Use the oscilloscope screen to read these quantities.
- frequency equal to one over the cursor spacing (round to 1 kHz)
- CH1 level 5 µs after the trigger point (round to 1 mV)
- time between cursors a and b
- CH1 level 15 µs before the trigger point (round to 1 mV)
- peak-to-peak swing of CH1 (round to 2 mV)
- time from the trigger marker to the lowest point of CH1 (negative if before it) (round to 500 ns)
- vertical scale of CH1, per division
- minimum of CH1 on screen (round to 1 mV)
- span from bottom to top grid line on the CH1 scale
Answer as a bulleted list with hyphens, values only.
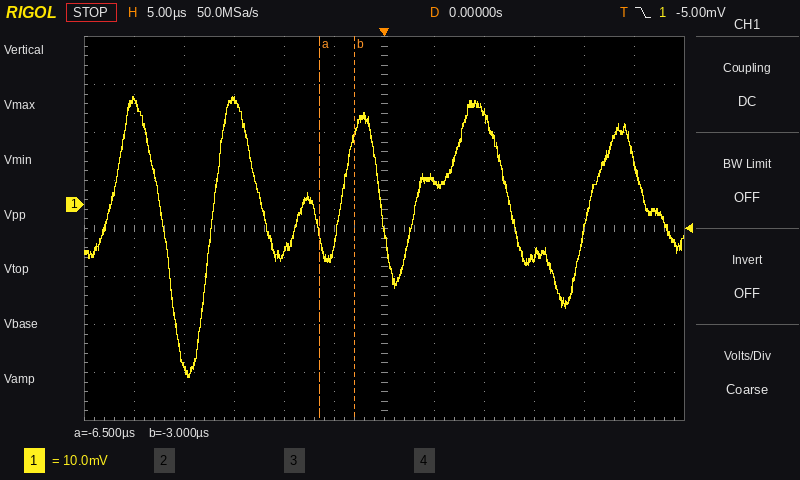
- 286 kHz
- 5 mV
- 3.5 µs
- 22 mV
- 58 mV
- -19.5 µs
- 10 mV
- -36 mV
- 80 mV
